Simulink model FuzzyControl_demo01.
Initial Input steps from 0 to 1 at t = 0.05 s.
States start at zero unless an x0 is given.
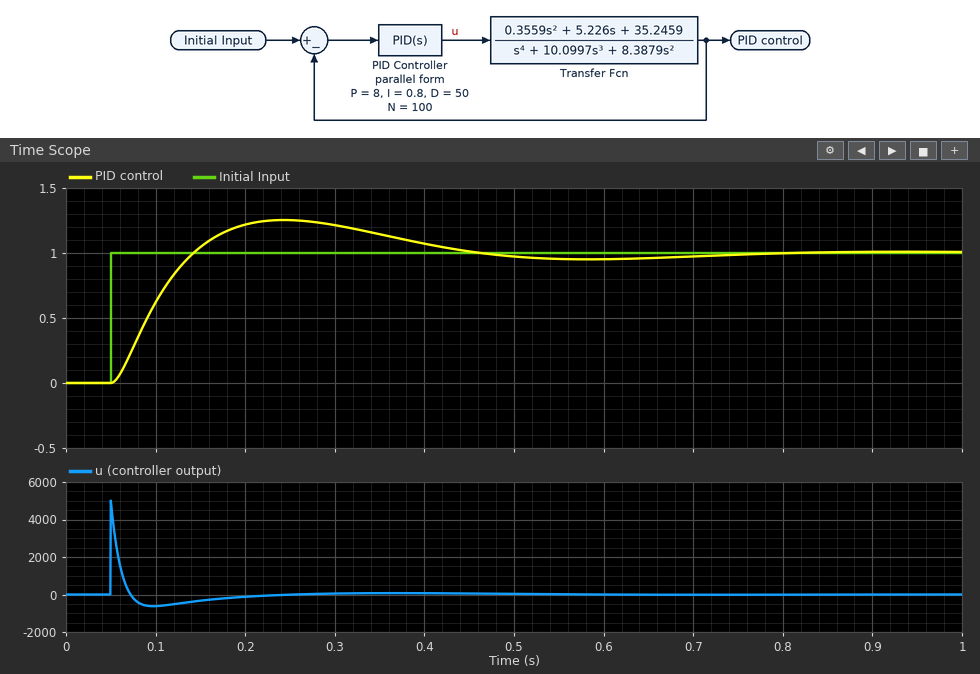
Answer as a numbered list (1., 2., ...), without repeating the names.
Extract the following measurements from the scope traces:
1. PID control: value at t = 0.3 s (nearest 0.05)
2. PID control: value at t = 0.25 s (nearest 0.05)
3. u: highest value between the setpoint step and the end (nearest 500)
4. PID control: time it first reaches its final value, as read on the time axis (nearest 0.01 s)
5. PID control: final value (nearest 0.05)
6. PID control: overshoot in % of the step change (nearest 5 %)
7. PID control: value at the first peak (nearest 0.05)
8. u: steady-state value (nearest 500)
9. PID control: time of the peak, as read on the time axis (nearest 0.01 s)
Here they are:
1. 1.20
2. 1.25
3. 5000
4. 0.14 s
5. 1.00
6. 25 %
7. 1.25
8. 0
9. 0.24 s
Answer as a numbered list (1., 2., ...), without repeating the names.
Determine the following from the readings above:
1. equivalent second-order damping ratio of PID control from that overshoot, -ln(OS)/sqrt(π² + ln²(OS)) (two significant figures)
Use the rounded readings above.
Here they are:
1. 0.40
